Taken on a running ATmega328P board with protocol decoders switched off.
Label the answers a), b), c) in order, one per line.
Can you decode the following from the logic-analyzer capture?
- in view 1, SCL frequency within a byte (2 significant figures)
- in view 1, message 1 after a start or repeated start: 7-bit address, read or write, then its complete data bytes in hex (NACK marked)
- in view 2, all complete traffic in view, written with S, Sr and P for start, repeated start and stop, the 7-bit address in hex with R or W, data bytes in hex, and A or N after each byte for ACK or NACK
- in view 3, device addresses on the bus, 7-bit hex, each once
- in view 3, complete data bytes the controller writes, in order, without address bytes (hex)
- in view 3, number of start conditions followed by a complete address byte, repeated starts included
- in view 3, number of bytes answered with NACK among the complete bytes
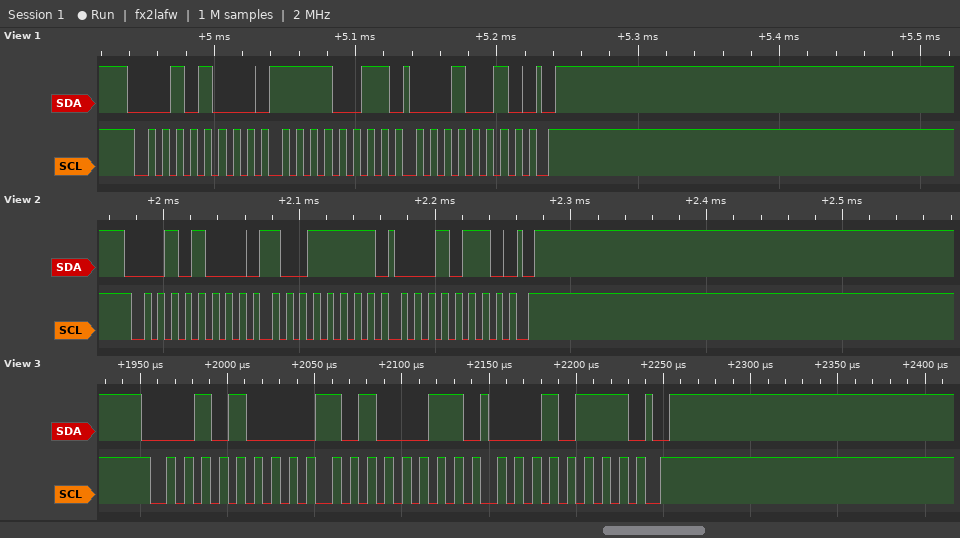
a) 100 kHz
b) 0x14 write: F3 12
c) S 14W A 9F A 16 A P
d) 0x14
e) A3 17
f) 1
g) 0
